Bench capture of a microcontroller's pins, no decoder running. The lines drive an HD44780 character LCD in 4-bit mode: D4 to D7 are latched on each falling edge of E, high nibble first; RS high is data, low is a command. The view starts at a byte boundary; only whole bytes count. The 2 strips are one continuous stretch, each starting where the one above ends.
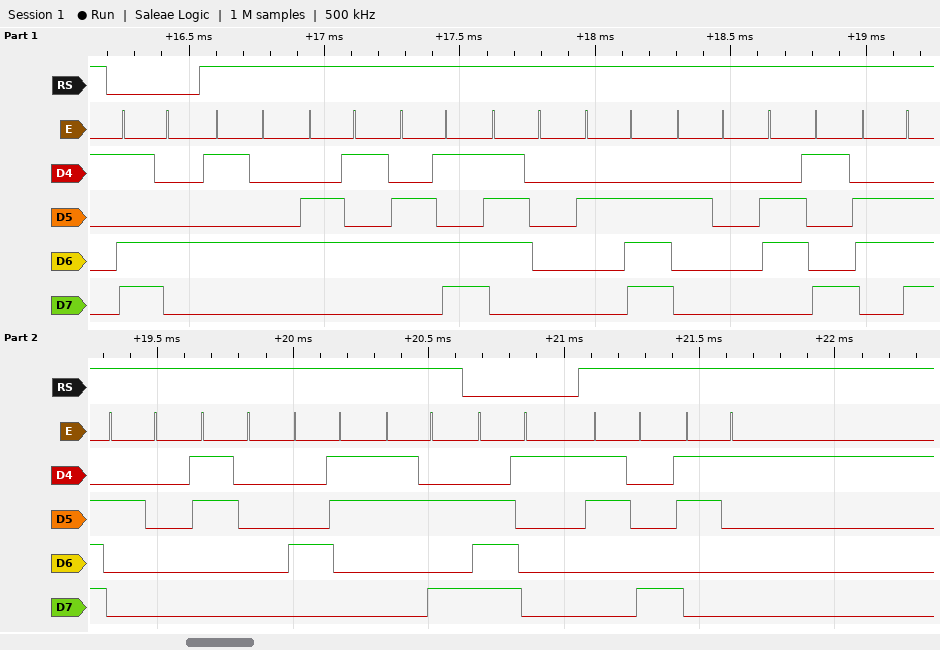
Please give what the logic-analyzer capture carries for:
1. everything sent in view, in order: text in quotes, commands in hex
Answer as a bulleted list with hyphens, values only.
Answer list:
- 0xD4 "Temp. in 0C:" 0xE1 "81"
